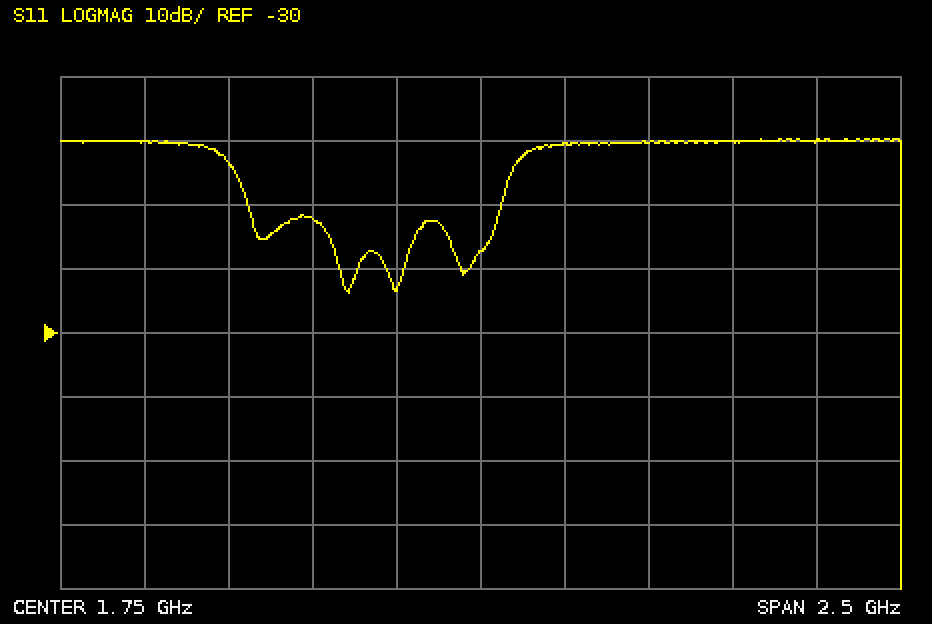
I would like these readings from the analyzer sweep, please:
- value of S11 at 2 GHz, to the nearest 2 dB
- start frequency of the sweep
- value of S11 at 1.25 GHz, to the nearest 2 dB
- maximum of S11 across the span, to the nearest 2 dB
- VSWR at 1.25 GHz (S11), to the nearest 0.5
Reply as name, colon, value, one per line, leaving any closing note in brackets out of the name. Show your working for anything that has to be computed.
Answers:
value of S11 at 2 GHz, to the nearest 2 dB: 0 dB
start frequency of the sweep: 500 MHz
value of S11 at 1.25 GHz, to the nearest 2 dB: -12 dB
maximum of S11 across the span, to the nearest 2 dB: 0 dB
VSWR at 1.25 GHz (S11), to the nearest 0.5: |Γ| = 10^(-12/20) = 0.2512; VSWR = (1 + 0.2512)/(1 − 0.2512) ≈ 1.67, so 1.5 to the nearest 0.5
